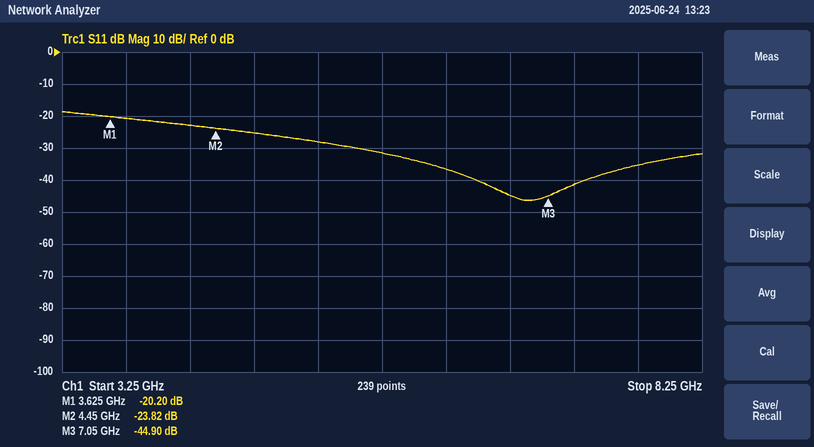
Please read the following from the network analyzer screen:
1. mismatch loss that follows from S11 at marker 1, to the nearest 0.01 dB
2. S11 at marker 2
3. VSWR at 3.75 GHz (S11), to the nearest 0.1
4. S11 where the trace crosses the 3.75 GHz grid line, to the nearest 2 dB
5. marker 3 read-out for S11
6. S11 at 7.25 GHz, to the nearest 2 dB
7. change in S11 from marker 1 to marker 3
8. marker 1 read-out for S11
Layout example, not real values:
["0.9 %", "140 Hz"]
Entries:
["0.04 dB", "-23.82 dB", "1.2", "-20 dB", "-44.90 dB", "-42 dB", "-24.70 dB", "-20.20 dB"]
